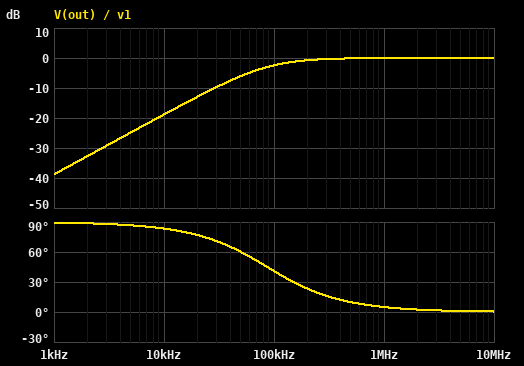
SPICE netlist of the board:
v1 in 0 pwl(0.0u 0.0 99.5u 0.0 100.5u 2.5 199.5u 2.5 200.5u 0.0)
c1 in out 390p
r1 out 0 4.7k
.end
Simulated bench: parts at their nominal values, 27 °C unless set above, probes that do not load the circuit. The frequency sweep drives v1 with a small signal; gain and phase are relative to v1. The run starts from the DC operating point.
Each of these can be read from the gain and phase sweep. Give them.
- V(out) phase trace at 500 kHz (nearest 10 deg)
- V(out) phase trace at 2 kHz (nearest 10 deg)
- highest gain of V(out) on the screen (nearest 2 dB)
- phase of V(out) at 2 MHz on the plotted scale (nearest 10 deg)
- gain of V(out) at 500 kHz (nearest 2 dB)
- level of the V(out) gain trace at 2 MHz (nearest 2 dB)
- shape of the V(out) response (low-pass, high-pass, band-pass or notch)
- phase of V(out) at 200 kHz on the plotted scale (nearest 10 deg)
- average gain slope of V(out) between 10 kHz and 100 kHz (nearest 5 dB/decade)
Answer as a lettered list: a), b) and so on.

a) 10 deg
b) 90 deg
c) 0 dB
d) 0 deg
e) 0 dB
f) 0 dB
g) high-pass
h) 20 deg
i) 15 dB/decade
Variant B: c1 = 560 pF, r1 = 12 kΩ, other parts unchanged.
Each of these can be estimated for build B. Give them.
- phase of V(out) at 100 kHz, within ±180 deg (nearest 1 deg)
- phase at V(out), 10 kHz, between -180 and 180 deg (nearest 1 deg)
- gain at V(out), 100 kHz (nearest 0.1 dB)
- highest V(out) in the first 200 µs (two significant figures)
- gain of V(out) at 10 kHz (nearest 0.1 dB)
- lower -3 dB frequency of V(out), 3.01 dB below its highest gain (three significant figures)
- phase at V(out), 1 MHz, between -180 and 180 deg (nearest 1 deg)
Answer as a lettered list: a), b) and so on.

a) 13 deg
b) 67 deg
c) -0.2 dB
d) 2.3 V
e) -8.2 dB
f) 23.7 kHz
g) 1 deg
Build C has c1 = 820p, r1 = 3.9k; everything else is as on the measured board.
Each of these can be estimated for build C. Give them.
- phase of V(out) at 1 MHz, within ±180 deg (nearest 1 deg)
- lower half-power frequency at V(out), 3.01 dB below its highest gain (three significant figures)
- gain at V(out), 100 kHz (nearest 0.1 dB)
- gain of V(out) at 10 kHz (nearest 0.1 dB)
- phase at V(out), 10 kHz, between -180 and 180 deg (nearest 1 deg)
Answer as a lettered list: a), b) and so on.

a) 3 deg
b) 49.8 kHz
c) -1.0 dB
d) -14.1 dB
e) 79 deg
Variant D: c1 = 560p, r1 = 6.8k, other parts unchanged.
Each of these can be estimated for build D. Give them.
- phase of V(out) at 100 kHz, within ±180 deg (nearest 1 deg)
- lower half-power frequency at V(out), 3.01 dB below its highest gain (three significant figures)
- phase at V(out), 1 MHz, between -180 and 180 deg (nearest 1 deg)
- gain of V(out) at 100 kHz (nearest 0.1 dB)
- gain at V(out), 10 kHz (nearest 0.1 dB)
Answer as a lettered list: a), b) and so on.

a) 23 deg
b) 41.8 kHz
c) 2 deg
d) -0.7 dB
e) -12.7 dB
